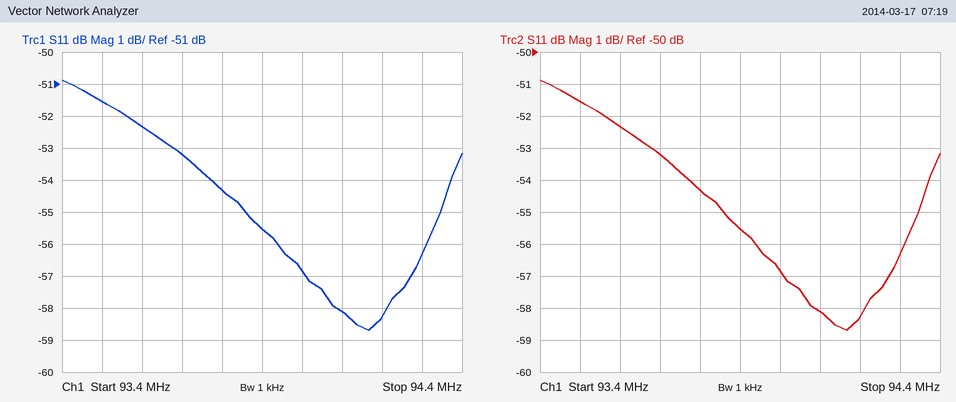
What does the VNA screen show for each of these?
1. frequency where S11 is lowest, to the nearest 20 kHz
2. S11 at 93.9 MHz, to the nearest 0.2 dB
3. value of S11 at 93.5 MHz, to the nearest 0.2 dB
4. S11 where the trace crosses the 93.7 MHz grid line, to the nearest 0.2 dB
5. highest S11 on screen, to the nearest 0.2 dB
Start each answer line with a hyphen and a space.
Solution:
- 94.16 MHz
- -55.6 dB
- -51.6 dB
- -53.2 dB
- -50.8 dB
